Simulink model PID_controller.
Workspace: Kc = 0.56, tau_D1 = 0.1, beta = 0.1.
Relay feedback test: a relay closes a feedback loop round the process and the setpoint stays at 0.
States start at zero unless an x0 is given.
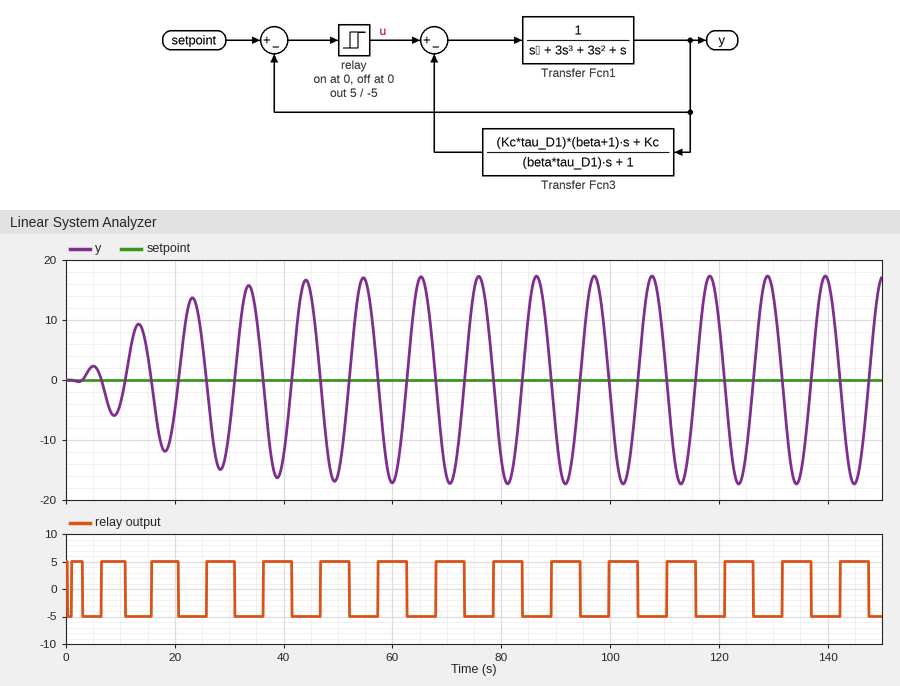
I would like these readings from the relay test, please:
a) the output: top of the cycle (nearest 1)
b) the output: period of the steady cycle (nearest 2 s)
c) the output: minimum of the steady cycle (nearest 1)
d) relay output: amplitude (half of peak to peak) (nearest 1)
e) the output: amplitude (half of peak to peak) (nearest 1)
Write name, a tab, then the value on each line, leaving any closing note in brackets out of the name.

the output: top of the cycle	17
the output: period of the steady cycle	10 s
the output: minimum of the steady cycle	-17
relay output: amplitude (half of peak to peak)	5
the output: amplitude (half of peak to peak)	17
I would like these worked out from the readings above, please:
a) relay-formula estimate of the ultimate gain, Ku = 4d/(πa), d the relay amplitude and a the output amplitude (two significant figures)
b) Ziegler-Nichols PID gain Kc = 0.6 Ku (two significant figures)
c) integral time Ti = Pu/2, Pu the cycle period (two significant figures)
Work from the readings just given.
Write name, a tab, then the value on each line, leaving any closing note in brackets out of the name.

relay-formula estimate of the ultimate gain, Ku = 4d/(πa), d the relay amplitude and a the output amplitude	0.37
Ziegler-Nichols PID gain Kc = 0.6 Ku	0.22
integral time Ti = Pu/2, Pu the cycle period	5.0 s
